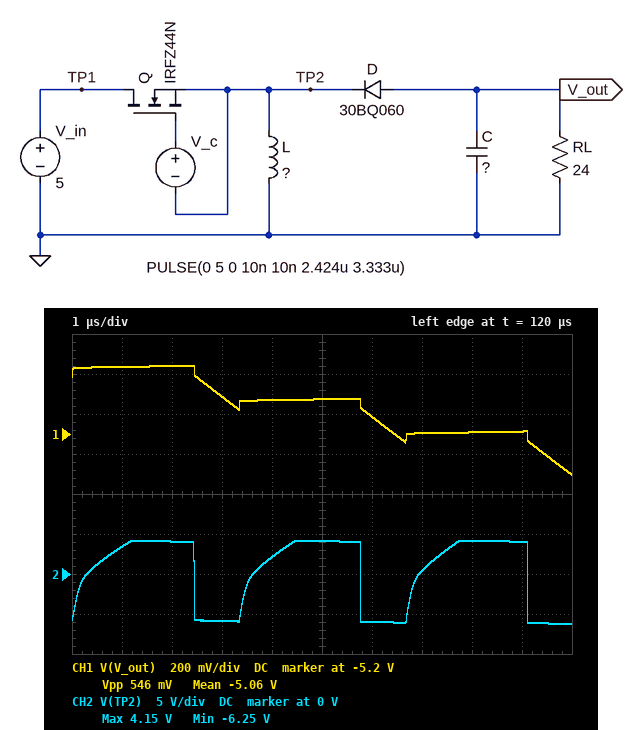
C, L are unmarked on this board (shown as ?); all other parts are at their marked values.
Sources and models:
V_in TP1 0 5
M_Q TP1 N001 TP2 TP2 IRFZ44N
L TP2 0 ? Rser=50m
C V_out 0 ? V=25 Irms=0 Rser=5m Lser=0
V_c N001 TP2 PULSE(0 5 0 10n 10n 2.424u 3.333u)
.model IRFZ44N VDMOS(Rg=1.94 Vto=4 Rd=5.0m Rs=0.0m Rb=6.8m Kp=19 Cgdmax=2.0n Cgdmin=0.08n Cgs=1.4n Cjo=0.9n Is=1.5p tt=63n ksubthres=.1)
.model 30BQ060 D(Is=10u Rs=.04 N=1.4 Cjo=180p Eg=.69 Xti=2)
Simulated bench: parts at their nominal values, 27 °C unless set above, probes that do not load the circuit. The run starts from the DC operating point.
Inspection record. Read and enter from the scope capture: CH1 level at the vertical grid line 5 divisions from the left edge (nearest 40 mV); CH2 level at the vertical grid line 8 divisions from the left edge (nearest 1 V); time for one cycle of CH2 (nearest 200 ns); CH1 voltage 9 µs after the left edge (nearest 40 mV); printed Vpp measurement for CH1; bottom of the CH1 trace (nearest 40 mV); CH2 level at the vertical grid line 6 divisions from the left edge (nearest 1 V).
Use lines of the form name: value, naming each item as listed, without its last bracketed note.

CH1 level at the vertical grid line 5 divisions from the left edge: -5.04 V
CH2 level at the vertical grid line 8 divisions from the left edge: 4 V
time for one cycle of CH2: 3.4 µs
CH1 voltage 9 µs after the left edge: -5.20 V
printed Vpp measurement for CH1: 546 mV
bottom of the CH1 trace: -5.40 V
CH2 level at the vertical grid line 6 divisions from the left edge: -6 V
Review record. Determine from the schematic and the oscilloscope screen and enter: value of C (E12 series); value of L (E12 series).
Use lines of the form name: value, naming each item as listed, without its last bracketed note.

value of C: 47 µF
value of L: 18 µH
